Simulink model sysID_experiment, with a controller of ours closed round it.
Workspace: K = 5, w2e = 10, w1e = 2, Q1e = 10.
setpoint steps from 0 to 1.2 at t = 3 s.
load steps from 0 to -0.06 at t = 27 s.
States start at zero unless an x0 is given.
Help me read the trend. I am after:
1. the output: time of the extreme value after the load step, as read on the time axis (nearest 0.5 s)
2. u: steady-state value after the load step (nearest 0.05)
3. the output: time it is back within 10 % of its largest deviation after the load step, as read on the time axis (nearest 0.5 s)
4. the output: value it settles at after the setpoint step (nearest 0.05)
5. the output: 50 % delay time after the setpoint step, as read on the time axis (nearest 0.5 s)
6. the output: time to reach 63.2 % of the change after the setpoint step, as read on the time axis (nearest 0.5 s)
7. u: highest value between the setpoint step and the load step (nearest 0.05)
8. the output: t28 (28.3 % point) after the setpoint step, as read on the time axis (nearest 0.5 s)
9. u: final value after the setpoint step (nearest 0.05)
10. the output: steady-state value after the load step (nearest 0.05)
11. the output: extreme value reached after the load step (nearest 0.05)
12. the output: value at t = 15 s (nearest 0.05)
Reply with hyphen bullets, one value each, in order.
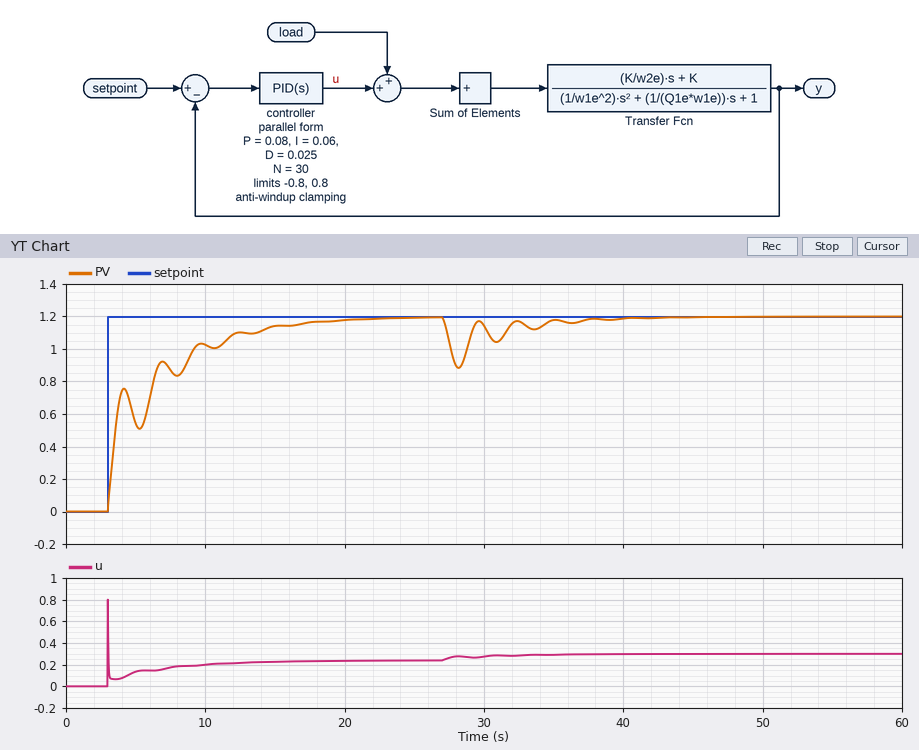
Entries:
- 28.0 s
- 0.30
- 37.0 s
- 1.20
- 3.5 s
- 6.0 s
- 0.80
- 3.5 s
- 0.25
- 1.20
- 0.90
- 1.15
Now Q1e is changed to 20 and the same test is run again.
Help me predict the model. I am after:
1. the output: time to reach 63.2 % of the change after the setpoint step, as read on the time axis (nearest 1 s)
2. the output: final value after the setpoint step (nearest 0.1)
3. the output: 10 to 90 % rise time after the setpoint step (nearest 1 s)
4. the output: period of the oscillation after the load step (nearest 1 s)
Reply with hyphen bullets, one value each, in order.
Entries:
- 4 s
- 1.2
- 9 s
- 3 s
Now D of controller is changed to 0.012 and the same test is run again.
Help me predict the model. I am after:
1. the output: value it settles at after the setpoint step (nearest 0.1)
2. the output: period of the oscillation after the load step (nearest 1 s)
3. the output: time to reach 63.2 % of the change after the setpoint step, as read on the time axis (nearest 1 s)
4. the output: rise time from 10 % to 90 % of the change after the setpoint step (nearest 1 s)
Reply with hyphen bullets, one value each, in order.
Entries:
- 1.2
- 3 s
- 4 s
- 6 s
